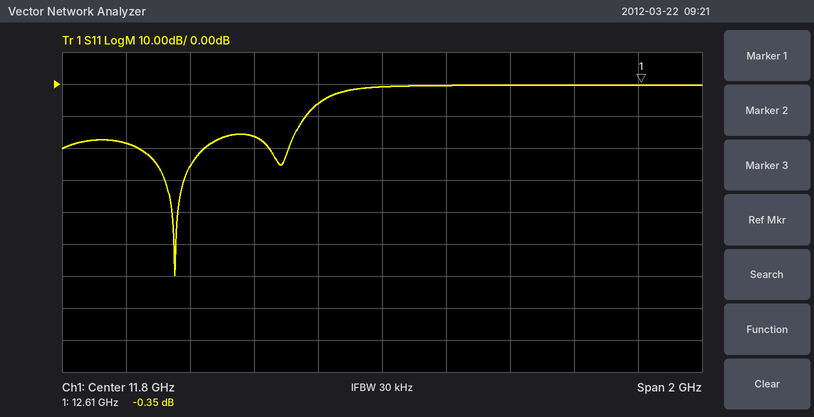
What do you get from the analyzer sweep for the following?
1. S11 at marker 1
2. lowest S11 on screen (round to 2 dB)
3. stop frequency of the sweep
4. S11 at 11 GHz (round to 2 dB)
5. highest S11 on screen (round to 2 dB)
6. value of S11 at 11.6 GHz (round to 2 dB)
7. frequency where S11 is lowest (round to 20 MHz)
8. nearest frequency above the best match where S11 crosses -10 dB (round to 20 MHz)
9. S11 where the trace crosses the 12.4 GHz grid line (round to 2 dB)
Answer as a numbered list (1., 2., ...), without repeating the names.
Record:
1. -0.35 dB
2. -60 dB
3. 12.8 GHz
4. -18 dB
5. 0 dB
6. -6 dB
7. 11.16 GHz
8. 11.56 GHz
9. 0 dB
